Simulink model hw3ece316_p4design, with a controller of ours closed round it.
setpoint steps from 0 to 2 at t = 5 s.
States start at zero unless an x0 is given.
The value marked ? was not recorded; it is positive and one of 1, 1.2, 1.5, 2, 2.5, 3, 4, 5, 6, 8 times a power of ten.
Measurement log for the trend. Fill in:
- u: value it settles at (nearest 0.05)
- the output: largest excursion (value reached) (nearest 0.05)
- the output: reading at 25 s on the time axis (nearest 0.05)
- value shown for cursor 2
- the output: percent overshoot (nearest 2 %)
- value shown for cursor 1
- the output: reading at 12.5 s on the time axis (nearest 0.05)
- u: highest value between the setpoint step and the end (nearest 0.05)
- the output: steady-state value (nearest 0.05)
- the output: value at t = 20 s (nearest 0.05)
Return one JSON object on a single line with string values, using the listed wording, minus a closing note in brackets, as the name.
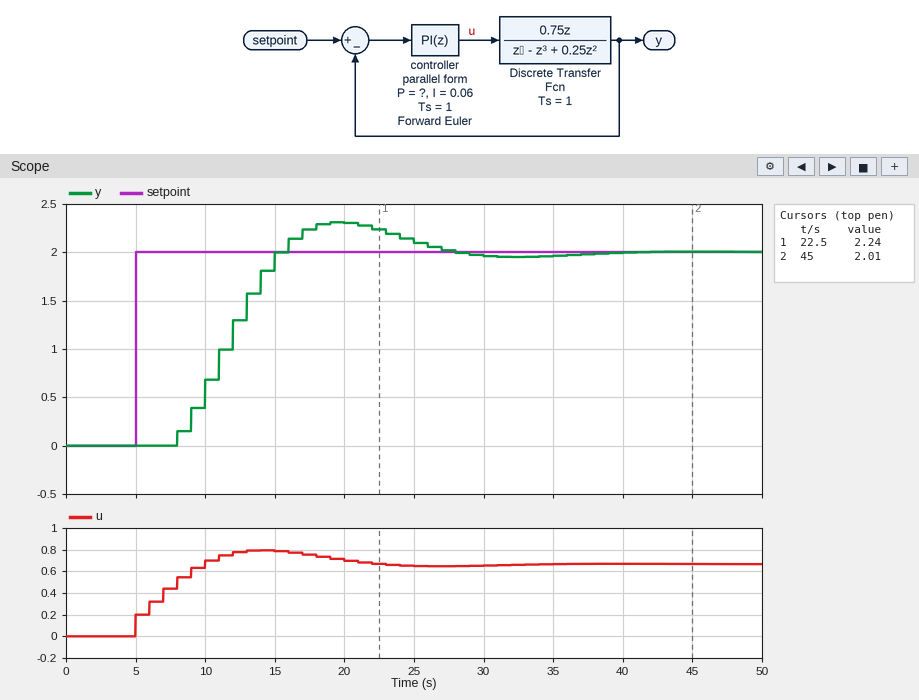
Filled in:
{"u: value it settles at": "0.65", "the output: largest excursion (value reached)": "2.30", "the output: reading at 25 s on the time axis": "2.10", "value shown for cursor 2": "2.01", "the output: percent overshoot": "16 %", "value shown for cursor 1": "2.24", "the output: reading at 12.5 s on the time axis": "1.30", "u: highest value between the setpoint step and the end": "0.80", "the output: steady-state value": "2.00", "the output: value at t = 20 s": "2.30"}
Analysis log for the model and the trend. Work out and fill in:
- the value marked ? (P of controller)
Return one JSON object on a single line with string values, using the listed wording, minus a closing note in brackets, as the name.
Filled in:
{"the value marked ?": "0.1"}
